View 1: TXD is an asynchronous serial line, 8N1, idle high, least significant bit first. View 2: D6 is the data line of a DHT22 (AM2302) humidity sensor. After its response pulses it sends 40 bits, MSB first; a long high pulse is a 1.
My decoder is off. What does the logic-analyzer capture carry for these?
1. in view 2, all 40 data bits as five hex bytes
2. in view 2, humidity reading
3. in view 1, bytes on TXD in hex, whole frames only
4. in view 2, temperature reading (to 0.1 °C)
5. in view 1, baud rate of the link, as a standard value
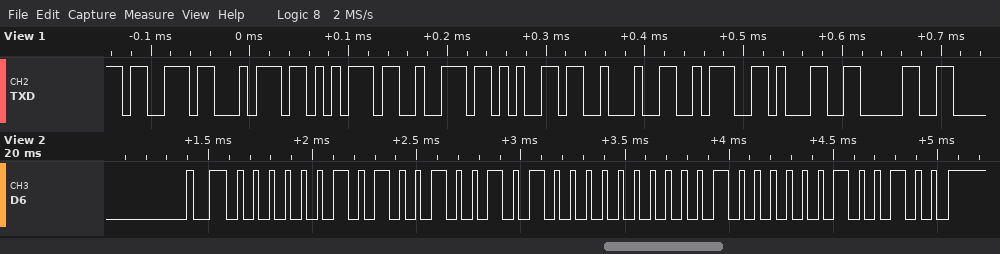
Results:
02 92 80 10 24
65.8 %
0x73 0x74 0x75 0x72 0x65 0x22 0x3A 0x31 0x30
-1.6 °C
115200 baud
